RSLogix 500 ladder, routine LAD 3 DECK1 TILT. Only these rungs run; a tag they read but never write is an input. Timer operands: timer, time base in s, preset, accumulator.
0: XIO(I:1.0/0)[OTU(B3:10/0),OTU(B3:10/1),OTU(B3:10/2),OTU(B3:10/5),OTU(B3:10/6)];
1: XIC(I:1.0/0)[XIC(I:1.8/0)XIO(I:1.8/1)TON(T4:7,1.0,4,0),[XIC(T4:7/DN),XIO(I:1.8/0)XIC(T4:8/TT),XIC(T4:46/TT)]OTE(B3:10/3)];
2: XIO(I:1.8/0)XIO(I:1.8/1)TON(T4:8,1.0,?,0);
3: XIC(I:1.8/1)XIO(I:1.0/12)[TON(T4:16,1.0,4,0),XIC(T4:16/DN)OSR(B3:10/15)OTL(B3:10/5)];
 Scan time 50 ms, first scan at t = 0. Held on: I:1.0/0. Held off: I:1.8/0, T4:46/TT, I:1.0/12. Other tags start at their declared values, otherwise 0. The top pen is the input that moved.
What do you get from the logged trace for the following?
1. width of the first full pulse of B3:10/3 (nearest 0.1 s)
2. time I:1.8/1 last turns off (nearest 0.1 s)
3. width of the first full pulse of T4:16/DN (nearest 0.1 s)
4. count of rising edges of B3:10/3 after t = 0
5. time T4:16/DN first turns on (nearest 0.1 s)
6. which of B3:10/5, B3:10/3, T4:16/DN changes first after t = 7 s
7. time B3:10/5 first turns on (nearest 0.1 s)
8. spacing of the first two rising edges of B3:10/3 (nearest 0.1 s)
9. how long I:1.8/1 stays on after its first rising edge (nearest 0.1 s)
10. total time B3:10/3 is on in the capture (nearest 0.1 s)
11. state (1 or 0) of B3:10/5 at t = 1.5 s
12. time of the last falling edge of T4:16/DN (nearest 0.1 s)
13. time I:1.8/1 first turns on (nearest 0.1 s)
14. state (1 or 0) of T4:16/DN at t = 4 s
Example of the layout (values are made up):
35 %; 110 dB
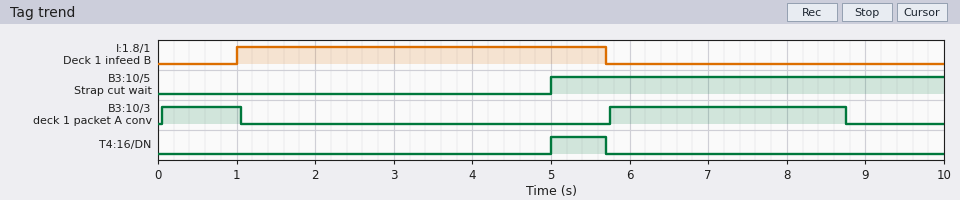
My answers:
1.0 s; 5.7 s; 0.7 s; 2; 5.0 s; B3:10/3; 5.0 s; 5.7 s; 4.7 s; 4.0 s; 0; 5.7 s; 1.0 s; 0
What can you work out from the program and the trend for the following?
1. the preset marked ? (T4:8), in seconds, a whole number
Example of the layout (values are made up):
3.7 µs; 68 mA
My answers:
3 s
